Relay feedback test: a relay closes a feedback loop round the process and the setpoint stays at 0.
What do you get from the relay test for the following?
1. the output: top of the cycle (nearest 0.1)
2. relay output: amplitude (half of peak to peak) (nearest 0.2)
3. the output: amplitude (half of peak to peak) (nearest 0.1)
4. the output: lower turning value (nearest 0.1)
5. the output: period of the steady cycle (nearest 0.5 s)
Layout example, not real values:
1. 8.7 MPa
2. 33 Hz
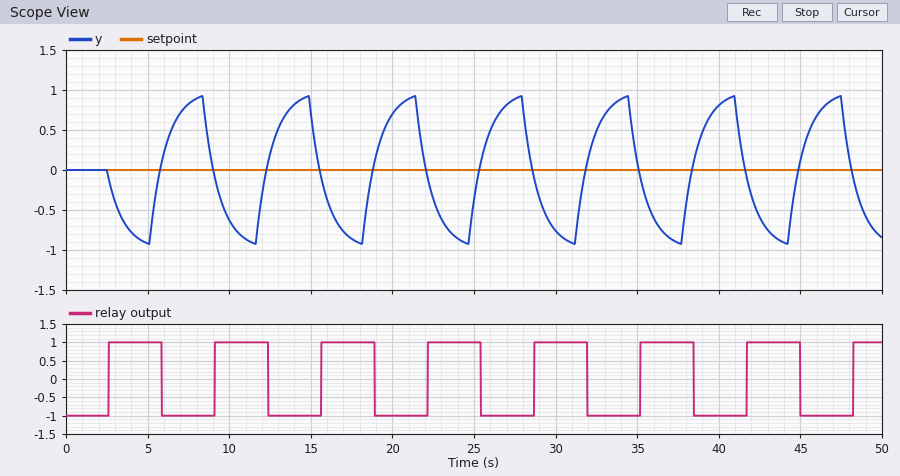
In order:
1. 0.9
2. 1.0
3. 0.9
4. -0.9
5. 6.5 s
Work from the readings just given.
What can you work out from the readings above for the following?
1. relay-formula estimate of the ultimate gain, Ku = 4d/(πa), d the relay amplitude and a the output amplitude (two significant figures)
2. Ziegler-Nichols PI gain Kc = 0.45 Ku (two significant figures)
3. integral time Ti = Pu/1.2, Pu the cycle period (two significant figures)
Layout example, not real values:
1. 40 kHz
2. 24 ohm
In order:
1. 1.4
2. 0.63
3. 5.4 s
